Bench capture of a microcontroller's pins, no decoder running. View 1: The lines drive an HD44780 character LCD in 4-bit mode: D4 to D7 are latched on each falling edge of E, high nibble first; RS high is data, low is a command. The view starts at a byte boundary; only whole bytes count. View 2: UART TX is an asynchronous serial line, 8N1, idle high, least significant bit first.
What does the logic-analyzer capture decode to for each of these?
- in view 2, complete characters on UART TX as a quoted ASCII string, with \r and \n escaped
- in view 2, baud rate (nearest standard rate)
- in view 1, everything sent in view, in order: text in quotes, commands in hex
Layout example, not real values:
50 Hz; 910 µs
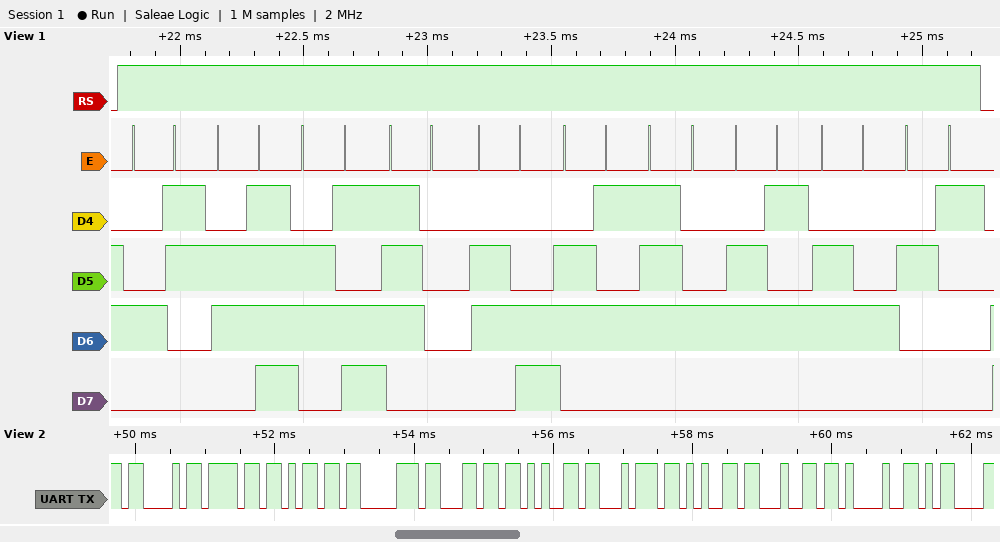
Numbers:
"Completed!\r"; 9600 baud; "Completed!"
